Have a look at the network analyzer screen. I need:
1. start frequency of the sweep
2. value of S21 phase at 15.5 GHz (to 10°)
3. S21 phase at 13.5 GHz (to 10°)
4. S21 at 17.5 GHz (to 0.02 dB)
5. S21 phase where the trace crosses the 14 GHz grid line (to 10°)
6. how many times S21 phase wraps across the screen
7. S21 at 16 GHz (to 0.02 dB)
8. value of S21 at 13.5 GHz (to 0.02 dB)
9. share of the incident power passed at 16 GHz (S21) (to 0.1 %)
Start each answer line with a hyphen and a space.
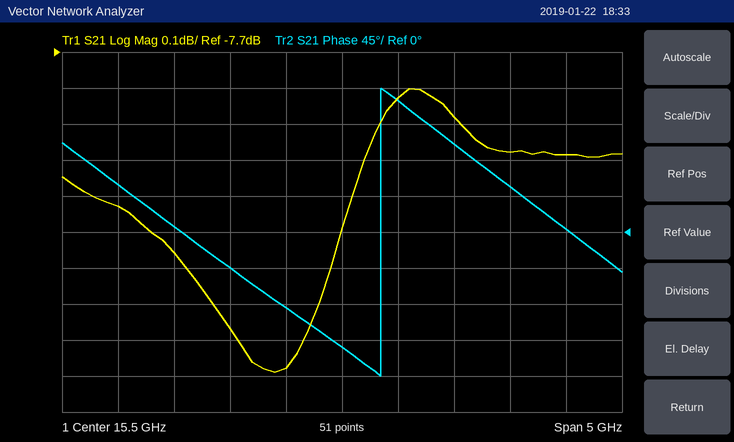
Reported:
- 13 GHz
- -140°
- 60°
- -7.98 dB
- 10°
- 1
- -7.82 dB
- -8.12 dB
- 16.5 %
